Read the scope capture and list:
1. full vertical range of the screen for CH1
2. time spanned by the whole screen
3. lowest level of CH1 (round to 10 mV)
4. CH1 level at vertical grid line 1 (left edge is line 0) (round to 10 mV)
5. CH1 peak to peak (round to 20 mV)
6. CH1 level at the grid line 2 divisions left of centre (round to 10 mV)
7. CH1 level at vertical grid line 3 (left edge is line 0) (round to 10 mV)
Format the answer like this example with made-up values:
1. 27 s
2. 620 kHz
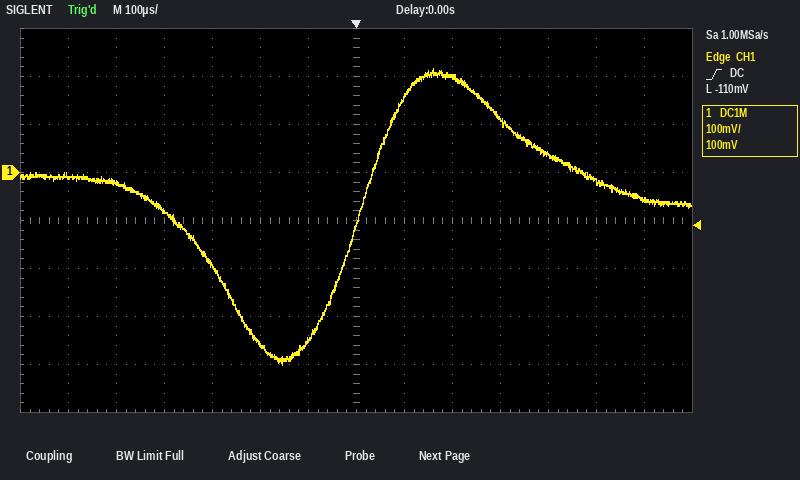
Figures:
1. 800 mV
2. 1.4 ms
3. -400 mV
4. -10 mV
5. 620 mV
6. -360 mV
7. -80 mV
